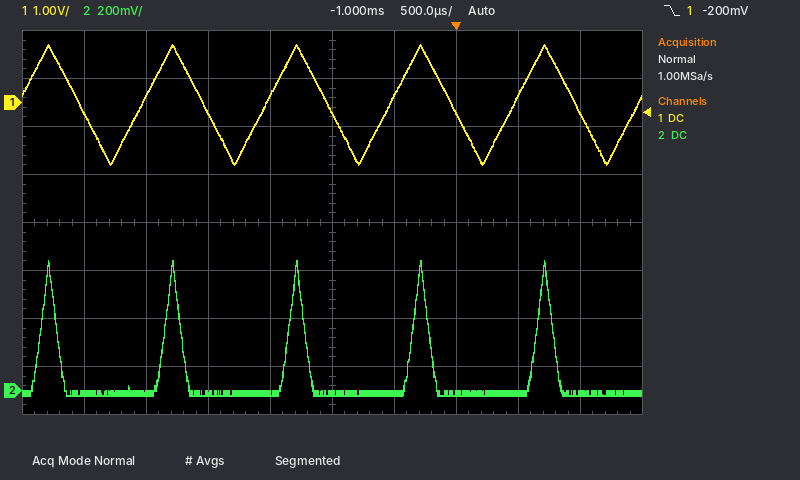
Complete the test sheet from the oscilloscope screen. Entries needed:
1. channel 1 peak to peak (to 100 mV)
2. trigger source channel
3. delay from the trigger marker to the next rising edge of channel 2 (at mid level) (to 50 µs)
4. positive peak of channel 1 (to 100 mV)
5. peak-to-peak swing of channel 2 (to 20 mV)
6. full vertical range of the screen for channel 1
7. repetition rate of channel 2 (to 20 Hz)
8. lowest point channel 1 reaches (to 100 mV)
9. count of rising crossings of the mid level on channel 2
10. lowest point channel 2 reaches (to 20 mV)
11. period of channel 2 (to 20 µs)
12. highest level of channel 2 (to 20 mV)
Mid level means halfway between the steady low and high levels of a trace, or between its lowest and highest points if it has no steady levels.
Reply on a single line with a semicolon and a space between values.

2.5 V; channel 1; 650 µs; 1.2 V; 560 mV; 8 V; 1.00 kHz; -1.3 V; 5; -20 mV; 1.00 ms; 540 mV
